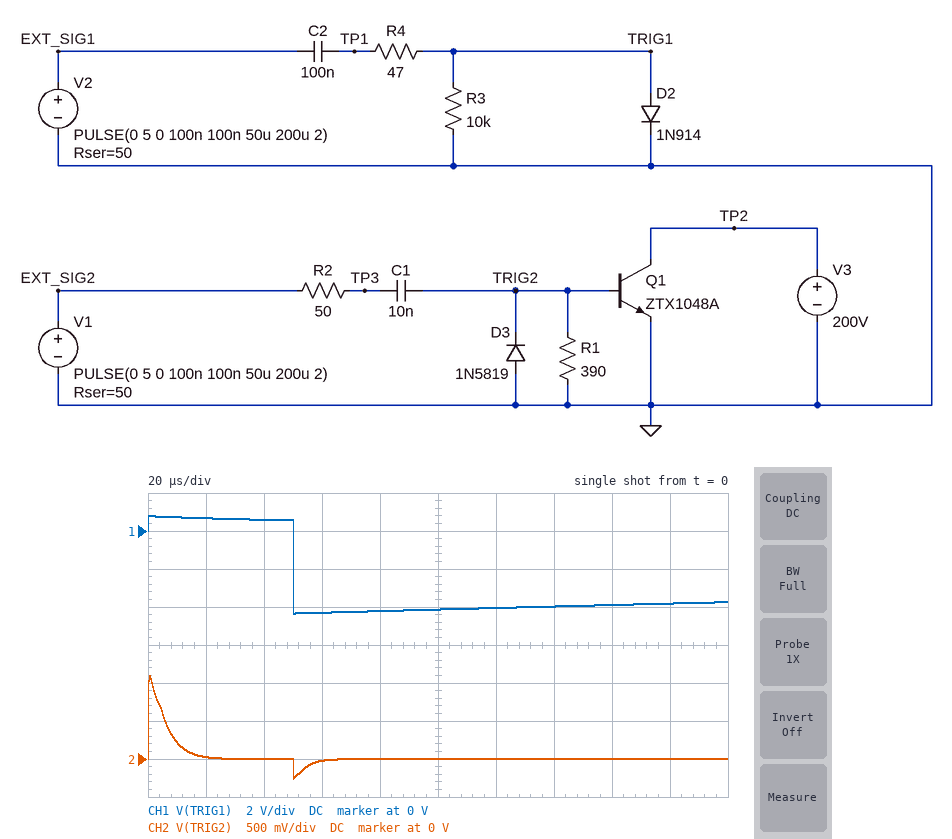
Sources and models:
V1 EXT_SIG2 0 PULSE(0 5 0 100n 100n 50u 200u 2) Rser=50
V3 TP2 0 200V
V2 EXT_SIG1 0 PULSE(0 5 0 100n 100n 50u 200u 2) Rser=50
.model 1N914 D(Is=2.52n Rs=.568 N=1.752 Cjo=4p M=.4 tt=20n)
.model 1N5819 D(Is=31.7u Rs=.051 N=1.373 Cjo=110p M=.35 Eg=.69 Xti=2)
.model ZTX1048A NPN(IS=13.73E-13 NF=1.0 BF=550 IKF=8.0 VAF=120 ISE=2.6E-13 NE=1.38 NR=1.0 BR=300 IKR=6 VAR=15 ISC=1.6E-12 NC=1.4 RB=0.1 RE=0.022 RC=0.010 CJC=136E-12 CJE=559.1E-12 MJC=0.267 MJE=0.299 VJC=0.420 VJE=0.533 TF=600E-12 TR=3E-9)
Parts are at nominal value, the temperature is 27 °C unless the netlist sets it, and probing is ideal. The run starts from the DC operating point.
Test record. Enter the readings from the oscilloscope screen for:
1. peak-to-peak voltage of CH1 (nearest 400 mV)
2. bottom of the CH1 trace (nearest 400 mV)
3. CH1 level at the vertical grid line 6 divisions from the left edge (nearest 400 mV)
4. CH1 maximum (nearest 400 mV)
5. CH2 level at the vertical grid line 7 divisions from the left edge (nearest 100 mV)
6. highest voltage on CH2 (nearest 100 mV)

5.2 V
-4.4 V
-4.0 V
800 mV
0 V
1.1 V
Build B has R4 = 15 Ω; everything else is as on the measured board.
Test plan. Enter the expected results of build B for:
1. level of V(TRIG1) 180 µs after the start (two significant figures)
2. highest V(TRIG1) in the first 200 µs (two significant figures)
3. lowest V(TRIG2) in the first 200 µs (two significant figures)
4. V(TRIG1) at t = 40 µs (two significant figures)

-3.9 V
810 mV
-260 mV
550 mV
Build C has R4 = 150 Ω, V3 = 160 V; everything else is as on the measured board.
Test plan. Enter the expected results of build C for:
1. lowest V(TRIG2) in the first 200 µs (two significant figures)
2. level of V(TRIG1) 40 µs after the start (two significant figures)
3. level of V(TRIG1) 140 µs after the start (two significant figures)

-260 mV
640 mV
-3.6 V
